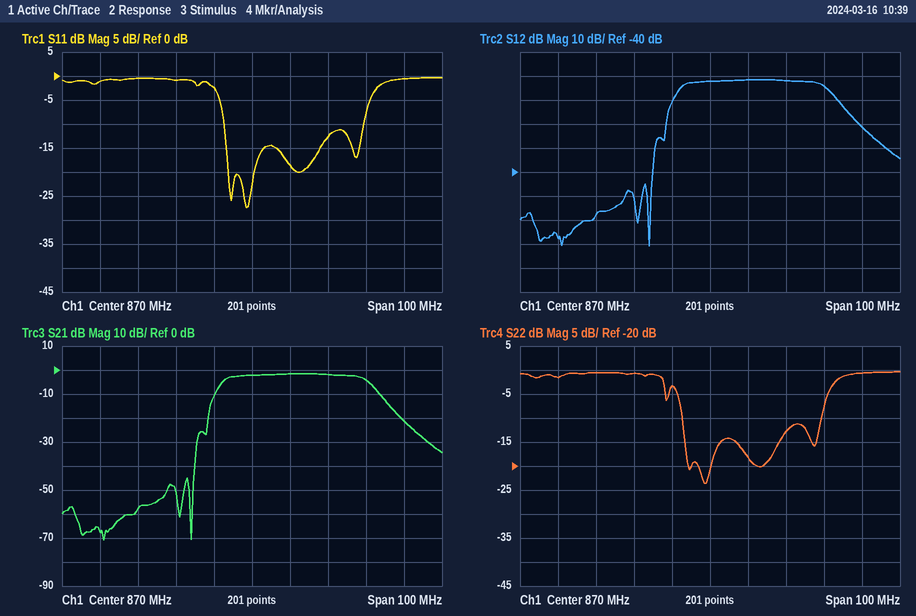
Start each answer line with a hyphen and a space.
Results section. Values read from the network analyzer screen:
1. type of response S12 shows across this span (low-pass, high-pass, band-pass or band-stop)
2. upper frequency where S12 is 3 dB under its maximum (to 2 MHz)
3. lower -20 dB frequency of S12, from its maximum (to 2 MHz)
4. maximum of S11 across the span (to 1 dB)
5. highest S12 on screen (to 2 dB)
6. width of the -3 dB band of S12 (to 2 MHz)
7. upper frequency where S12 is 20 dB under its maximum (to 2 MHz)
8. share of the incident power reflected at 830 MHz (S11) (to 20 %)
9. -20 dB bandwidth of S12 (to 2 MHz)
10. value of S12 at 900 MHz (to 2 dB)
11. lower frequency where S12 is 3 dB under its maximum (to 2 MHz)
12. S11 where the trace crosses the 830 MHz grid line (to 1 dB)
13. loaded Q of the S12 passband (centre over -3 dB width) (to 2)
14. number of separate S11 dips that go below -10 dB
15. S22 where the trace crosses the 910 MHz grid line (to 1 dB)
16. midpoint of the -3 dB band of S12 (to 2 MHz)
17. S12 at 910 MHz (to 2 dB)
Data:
- band-pass
- 900 MHz
- 858 MHz
- 0 dB
- -2 dB
- 38 MHz
- 910 MHz
- 80 %
- 52 MHz
- -4 dB
- 862 MHz
- -1 dB
- 24
- 4
- -1 dB
- 882 MHz
- -22 dB
